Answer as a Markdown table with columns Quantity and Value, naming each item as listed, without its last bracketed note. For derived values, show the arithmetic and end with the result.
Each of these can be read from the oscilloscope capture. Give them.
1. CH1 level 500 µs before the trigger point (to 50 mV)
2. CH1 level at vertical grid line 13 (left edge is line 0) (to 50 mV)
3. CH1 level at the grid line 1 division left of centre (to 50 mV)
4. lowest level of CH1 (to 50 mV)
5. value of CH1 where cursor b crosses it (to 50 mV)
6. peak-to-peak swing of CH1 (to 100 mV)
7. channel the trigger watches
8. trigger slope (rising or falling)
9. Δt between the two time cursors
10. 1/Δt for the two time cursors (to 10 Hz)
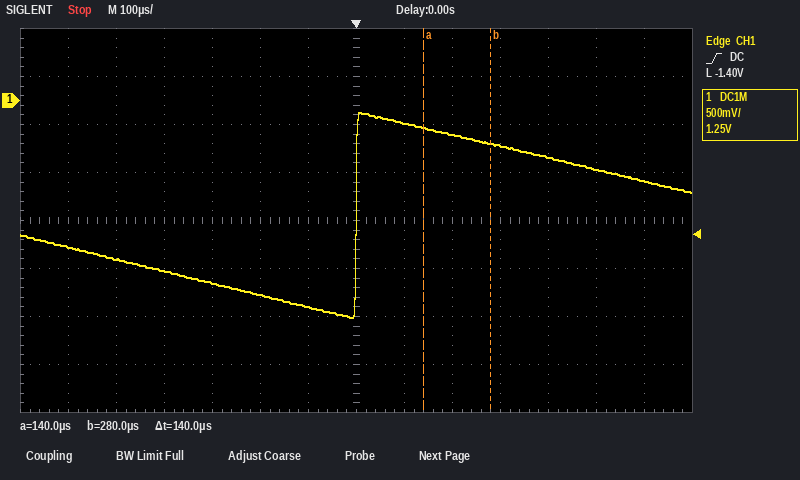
| Quantity | Value |
|---|---|
| CH1 level 500 µs before the trigger point | -1.65 V |
| CH1 level at vertical grid line 13 (left edge is line 0) | -850 mV |
| CH1 level at the grid line 1 division left of centre | -2.15 V |
| lowest level of CH1 | -2.25 V |
| value of CH1 where cursor b crosses it | -450 mV |
| peak-to-peak swing of CH1 | 2.10 V |
| channel the trigger watches | CH1 |
| trigger slope | rising |
| Δt between the two time cursors | 140 µs |
| 1/Δt for the two time cursors | 1 / 140 µs ≈ 7.14 kHz |
